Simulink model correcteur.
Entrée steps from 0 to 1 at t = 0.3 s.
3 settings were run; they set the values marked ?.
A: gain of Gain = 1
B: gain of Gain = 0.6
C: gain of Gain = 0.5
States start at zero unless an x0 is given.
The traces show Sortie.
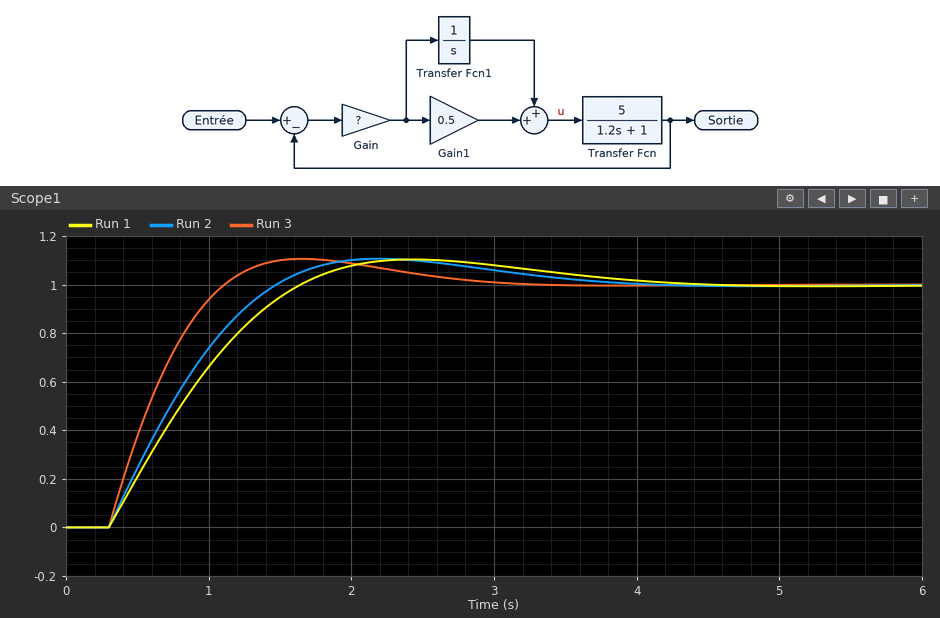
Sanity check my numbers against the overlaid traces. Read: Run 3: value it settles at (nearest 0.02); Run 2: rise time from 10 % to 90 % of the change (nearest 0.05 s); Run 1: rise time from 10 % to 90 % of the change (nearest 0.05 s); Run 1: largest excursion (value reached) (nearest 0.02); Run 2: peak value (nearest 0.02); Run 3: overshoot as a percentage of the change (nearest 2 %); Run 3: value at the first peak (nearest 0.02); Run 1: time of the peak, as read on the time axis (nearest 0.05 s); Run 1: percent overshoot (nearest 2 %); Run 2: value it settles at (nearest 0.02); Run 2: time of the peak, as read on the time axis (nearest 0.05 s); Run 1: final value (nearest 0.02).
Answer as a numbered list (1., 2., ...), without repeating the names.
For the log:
1. 1.00
2. 0.85 s
3. 1.00 s
4. 1.10
5. 1.10
6. 10 %
7. 1.10
8. 2.45 s
9. 10 %
10. 1.00
11. 2.20 s
12. 1.00
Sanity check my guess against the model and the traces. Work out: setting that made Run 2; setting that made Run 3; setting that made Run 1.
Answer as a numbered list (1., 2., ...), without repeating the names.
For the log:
1. B
2. A
3. C
